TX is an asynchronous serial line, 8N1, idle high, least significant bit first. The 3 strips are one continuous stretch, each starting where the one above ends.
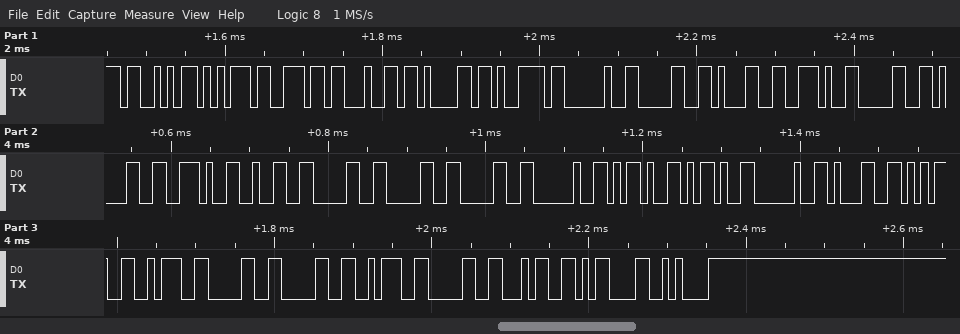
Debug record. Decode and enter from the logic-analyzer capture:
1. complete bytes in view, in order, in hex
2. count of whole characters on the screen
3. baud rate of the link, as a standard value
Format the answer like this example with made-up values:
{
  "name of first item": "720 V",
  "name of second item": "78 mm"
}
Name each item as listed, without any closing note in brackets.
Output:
{
  "complete bytes in view, in order, in hex": "0x53 0x75 0x6E 0x64 0x61 0x79 0x20 0x30 0x31 0x2E 0x30 0x31 0x2E 0x32 0x30 0x30 0x30 0x20 0x2D 0x2D 0x20 0x31 0x35 0x3A 0x30 0x30 0x3A 0x30 0x34 0x0D 0x0A",
  "count of whole characters on the screen": "31",
  "baud rate of the link, as a standard value": "115200 baud"
}
